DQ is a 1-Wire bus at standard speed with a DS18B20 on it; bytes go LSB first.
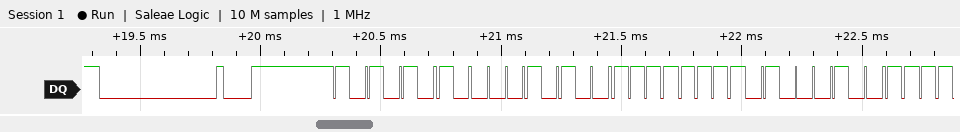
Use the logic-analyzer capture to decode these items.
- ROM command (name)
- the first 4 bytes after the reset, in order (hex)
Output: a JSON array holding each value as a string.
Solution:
["Match ROM", "55 28 FF 22"]
